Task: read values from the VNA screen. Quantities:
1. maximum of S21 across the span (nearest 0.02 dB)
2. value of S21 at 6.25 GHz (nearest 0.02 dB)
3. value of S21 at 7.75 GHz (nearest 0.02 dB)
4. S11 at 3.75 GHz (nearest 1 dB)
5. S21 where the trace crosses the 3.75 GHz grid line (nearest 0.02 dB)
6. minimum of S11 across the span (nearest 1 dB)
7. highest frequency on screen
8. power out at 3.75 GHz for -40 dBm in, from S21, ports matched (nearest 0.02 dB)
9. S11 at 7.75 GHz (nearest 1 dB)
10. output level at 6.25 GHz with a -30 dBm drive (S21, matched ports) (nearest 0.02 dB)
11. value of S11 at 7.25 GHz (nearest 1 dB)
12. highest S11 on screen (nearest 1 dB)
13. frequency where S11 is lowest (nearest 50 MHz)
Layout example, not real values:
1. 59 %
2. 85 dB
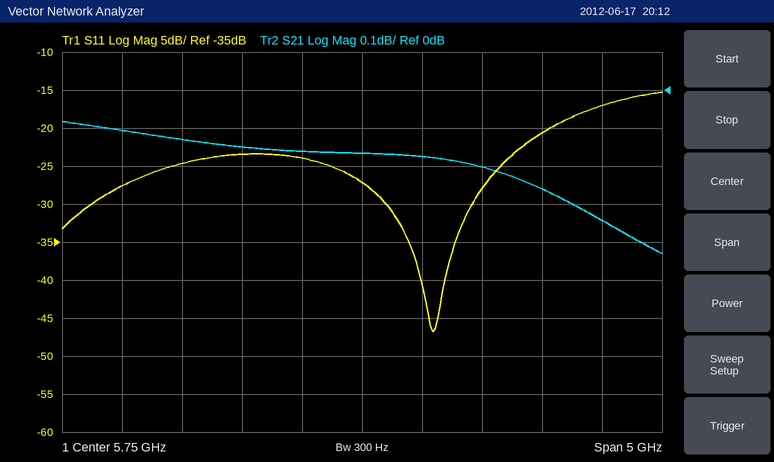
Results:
1. -0.08 dB
2. -0.18 dB
3. -0.34 dB
4. -28 dB
5. -0.10 dB
6. -47 dB
7. 8.25 GHz
8. -40.10 dBm
9. -17 dB
10. -30.18 dBm
11. -21 dB
12. -15 dB
13. 6.35 GHz
